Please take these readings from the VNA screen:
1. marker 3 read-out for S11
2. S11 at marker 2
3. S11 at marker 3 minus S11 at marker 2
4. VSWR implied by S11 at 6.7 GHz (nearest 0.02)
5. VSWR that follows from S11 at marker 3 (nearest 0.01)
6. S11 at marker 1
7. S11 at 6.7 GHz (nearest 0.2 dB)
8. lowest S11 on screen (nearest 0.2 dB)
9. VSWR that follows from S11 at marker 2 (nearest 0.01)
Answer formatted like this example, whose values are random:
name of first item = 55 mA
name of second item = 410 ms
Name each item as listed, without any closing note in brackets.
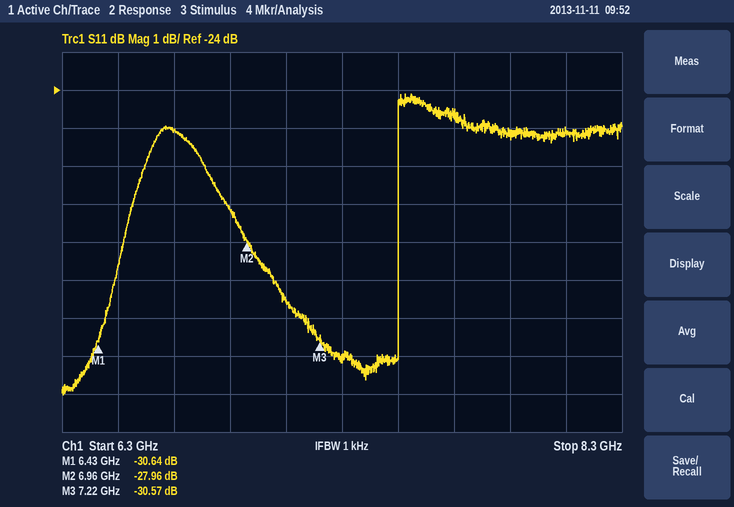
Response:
marker 3 read-out for S11 = -30.57 dB
S11 at marker 2 = -27.96 dB
S11 at marker 3 minus S11 at marker 2 = -2.61 dB
VSWR implied by S11 at 6.7 GHz = 1.12
VSWR that follows from S11 at marker 3 = 1.06
S11 at marker 1 = -30.64 dB
S11 at 6.7 GHz = -25.0 dB
lowest S11 on screen = -32.0 dB
VSWR that follows from S11 at marker 2 = 1.08
